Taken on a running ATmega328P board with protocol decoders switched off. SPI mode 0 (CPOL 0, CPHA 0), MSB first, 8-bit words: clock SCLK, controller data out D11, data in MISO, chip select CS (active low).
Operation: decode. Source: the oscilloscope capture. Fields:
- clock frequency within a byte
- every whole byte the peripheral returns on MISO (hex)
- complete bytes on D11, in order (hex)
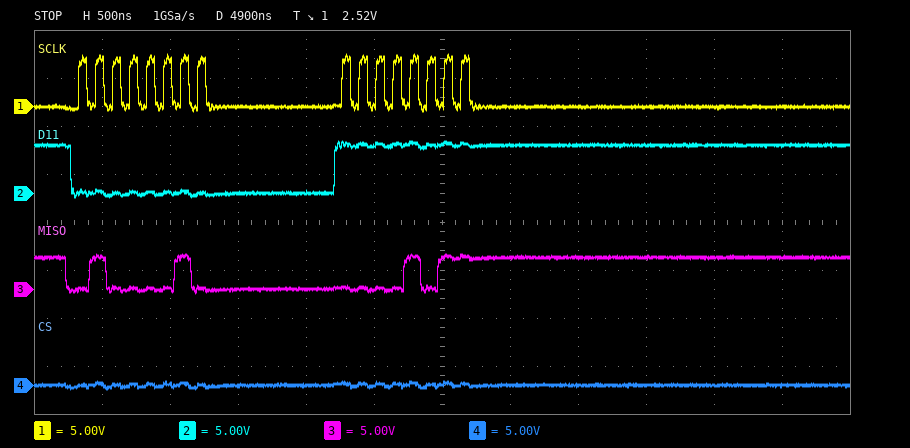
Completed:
8 MHz
42 0B
00 FF
